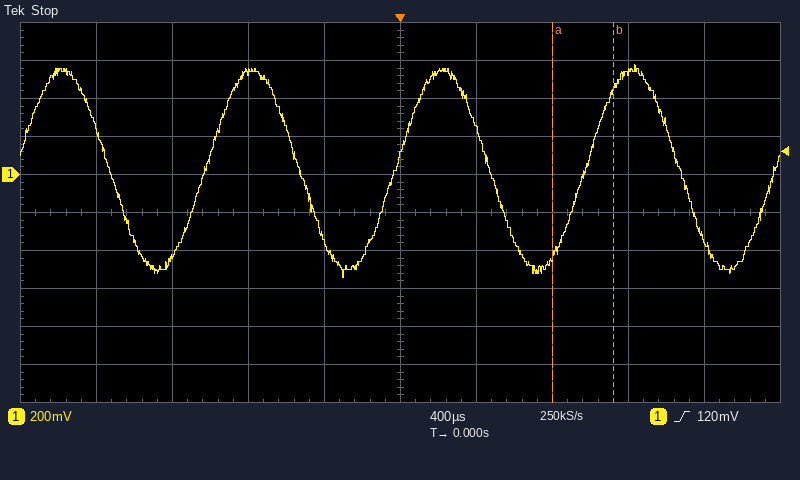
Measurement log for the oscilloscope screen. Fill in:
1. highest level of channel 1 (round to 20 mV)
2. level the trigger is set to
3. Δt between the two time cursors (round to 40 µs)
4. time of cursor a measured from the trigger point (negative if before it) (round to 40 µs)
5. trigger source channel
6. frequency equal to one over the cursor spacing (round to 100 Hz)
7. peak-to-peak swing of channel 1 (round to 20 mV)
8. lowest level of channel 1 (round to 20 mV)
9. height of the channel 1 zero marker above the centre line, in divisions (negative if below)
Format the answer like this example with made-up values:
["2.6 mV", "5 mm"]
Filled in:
["580 mV", "120 mV", "320 µs", "+800 µs", "channel 1", "3.1 kHz", "1.12 V", "-540 mV", "+1.0 div"]
